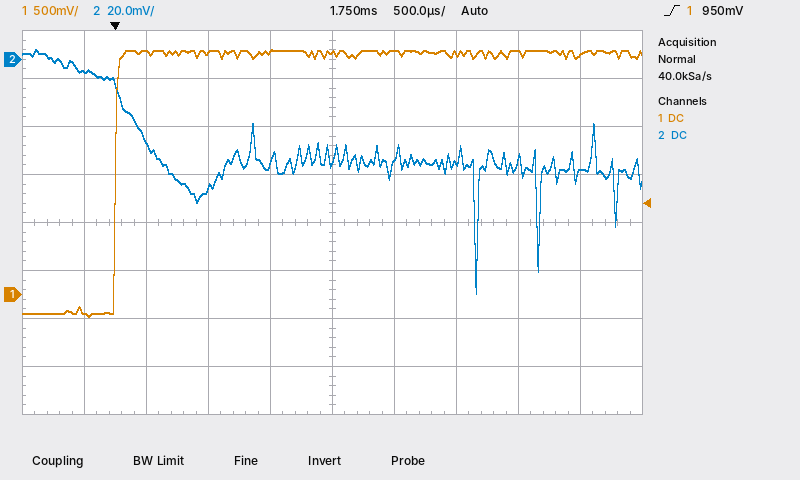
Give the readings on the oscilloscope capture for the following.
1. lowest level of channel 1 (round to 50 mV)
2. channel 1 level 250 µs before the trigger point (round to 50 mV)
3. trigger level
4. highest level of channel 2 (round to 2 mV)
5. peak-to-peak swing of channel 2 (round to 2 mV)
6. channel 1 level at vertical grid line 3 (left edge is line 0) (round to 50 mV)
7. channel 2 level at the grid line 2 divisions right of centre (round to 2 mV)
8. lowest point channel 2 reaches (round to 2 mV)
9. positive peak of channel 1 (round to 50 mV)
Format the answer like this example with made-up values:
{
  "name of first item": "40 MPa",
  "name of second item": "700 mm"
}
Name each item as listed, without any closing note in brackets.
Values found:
{
  "lowest level of channel 1": "-250 mV",
  "channel 1 level 250 µs before the trigger point": "-200 mV",
  "trigger level": "950 mV",
  "highest level of channel 2": "4 mV",
  "peak-to-peak swing of channel 2": "102 mV",
  "channel 1 level at vertical grid line 3 (left edge is line 0)": "2.50 V",
  "channel 2 level at the grid line 2 divisions right of centre": "-42 mV",
  "lowest point channel 2 reaches": "-98 mV",
  "positive peak of channel 1": "2.55 V"
}
